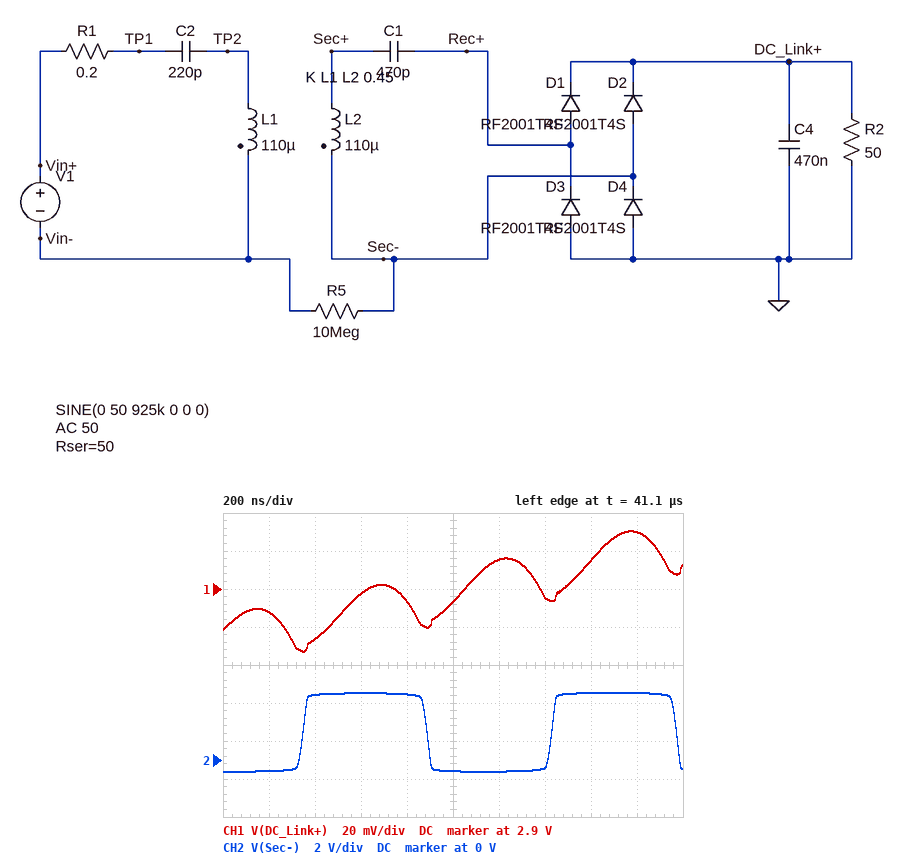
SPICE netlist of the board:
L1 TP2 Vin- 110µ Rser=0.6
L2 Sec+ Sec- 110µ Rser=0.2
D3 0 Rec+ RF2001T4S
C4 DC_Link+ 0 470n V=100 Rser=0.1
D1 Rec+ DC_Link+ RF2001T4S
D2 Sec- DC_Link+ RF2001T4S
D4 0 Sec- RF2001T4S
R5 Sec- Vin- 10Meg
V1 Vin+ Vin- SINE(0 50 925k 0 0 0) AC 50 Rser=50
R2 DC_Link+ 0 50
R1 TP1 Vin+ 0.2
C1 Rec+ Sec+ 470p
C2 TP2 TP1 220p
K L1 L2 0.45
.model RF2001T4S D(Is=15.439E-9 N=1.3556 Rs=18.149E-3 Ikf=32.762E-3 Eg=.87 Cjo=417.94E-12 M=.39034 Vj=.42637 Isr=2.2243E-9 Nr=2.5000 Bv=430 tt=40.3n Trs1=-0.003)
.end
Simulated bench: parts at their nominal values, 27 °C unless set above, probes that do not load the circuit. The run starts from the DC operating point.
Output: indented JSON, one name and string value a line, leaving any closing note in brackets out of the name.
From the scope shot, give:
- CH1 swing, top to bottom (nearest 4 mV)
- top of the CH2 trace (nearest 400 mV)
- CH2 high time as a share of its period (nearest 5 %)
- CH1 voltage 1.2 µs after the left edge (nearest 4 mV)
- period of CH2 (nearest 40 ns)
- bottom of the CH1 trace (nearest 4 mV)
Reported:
{
  "CH1 swing, top to bottom": "64 mV",
  "top of the CH2 trace": "3.6 V",
  "CH2 high time as a share of its period": "50 %",
  "CH1 voltage 1.2 µs after the left edge": "2.916 V",
  "period of CH2": "1.08 µs",
  "bottom of the CH1 trace": "2.868 V"
}
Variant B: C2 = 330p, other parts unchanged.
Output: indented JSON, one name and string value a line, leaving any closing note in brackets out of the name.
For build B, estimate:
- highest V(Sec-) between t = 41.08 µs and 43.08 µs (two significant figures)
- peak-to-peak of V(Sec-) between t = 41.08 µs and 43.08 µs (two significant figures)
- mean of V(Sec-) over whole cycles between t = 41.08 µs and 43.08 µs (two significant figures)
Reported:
{
  "highest V(Sec-) between t = 41.08 µs and 43.08 µs": "7.1 V",
  "peak-to-peak of V(Sec-) between t = 41.08 µs and 43.08 µs": "7.8 V",
  "mean of V(Sec-) over whole cycles between t = 41.08 µs and 43.08 µs": "3.2 V"
}
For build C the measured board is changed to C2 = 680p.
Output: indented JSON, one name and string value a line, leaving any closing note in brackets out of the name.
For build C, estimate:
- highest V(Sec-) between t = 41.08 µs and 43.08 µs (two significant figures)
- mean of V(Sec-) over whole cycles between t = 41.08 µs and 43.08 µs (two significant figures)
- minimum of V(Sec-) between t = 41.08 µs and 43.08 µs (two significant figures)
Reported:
{
  "highest V(Sec-) between t = 41.08 µs and 43.08 µs": "13 V",
  "mean of V(Sec-) over whole cycles between t = 41.08 µs and 43.08 µs": "5.9 V",
  "minimum of V(Sec-) between t = 41.08 µs and 43.08 µs": "-710 mV"
}
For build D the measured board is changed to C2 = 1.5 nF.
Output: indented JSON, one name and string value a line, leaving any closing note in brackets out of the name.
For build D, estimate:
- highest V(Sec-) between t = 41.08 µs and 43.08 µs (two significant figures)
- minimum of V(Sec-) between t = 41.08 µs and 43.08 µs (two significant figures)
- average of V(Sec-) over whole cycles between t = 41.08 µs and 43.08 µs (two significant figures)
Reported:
{
  "highest V(Sec-) between t = 41.08 µs and 43.08 µs": "6.6 V",
  "minimum of V(Sec-) between t = 41.08 µs and 43.08 µs": "-660 mV",
  "average of V(Sec-) over whole cycles between t = 41.08 µs and 43.08 µs": "2.9 V"
}
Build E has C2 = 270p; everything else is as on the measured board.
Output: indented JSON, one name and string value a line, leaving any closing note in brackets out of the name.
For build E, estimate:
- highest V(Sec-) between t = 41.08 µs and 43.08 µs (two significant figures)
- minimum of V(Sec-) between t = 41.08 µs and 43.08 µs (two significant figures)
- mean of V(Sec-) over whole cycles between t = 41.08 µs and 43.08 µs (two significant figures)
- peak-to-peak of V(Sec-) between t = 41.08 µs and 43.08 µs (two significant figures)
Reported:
{
  "highest V(Sec-) between t = 41.08 µs and 43.08 µs": "4.9 V",
  "minimum of V(Sec-) between t = 41.08 µs and 43.08 µs": "-640 mV",
  "mean of V(Sec-) over whole cycles between t = 41.08 µs and 43.08 µs": "2.1 V",
  "peak-to-peak of V(Sec-) between t = 41.08 µs and 43.08 µs": "5.5 V"
}
